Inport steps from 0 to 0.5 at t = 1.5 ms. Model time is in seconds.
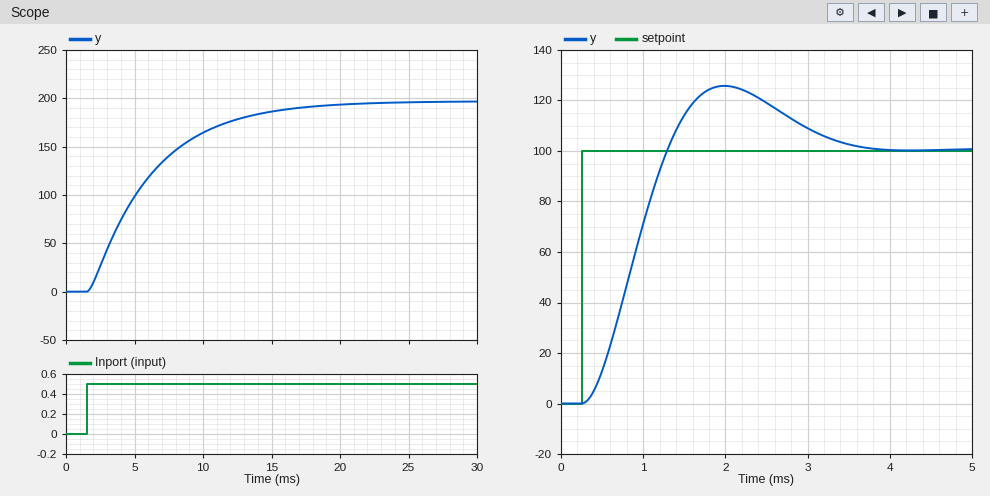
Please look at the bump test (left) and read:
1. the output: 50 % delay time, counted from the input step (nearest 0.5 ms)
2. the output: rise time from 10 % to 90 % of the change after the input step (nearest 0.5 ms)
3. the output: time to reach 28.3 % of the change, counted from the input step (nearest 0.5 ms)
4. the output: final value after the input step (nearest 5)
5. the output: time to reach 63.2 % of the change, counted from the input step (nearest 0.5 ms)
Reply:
3.5 ms
10.0 ms
2.0 ms
195
5.0 ms
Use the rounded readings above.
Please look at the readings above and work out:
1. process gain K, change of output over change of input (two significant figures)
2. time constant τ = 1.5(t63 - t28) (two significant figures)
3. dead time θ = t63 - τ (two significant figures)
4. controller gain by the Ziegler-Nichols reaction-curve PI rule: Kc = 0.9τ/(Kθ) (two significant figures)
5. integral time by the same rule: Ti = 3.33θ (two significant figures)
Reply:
390
4.5 ms
0.50 ms
0.021
1.7 ms
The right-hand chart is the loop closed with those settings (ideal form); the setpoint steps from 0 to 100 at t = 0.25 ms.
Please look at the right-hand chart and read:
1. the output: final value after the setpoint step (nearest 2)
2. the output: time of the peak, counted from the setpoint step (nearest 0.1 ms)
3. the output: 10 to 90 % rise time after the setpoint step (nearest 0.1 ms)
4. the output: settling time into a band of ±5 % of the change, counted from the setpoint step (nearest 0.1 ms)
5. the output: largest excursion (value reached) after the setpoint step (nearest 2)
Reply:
100
1.7 ms
0.7 ms
3.0 ms
126
